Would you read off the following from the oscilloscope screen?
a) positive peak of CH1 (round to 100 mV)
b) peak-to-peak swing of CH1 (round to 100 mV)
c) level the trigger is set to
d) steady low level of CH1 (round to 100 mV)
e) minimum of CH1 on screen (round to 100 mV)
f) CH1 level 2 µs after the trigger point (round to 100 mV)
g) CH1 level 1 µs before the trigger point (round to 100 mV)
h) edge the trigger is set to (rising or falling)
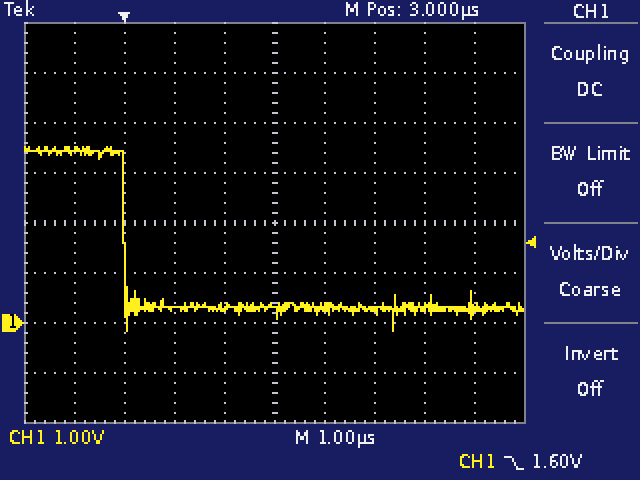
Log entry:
3.5 V
3.7 V
1.60 V
300 mV
-200 mV
300 mV
3.4 V
falling
